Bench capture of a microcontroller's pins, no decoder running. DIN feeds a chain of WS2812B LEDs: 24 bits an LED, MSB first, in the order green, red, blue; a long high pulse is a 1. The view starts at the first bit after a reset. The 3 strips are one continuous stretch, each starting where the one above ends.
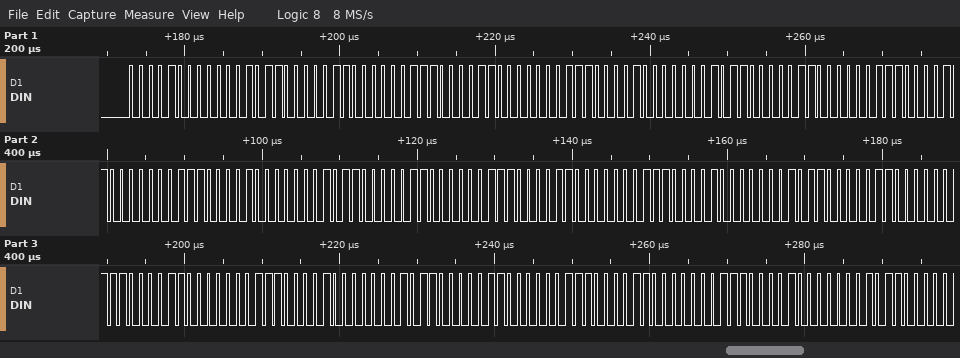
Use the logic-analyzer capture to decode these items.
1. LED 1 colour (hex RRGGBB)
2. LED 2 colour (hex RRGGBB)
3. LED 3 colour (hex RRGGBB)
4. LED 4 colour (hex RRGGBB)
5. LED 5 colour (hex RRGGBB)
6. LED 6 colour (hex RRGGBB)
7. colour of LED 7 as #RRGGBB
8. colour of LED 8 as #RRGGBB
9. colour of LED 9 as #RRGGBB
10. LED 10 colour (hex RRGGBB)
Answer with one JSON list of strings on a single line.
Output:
["#0B0806", "#0C0707", "#0B0806", "#0C0707", "#0B0806", "#0C0707", "#0B0806", "#0C0707", "#0B0806", "#0C0707"]
